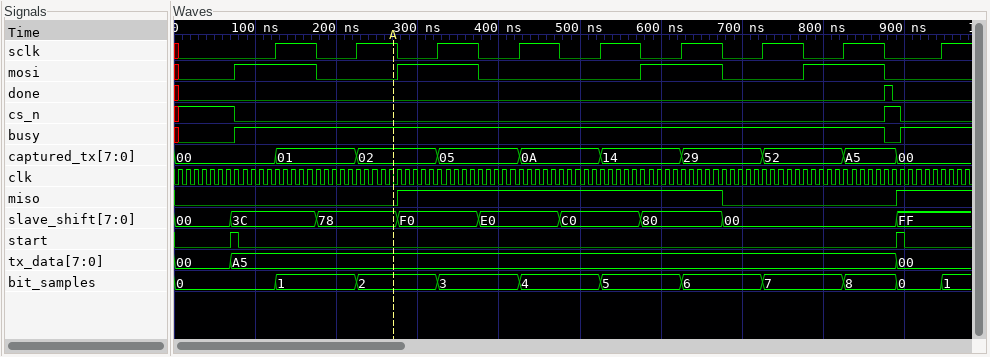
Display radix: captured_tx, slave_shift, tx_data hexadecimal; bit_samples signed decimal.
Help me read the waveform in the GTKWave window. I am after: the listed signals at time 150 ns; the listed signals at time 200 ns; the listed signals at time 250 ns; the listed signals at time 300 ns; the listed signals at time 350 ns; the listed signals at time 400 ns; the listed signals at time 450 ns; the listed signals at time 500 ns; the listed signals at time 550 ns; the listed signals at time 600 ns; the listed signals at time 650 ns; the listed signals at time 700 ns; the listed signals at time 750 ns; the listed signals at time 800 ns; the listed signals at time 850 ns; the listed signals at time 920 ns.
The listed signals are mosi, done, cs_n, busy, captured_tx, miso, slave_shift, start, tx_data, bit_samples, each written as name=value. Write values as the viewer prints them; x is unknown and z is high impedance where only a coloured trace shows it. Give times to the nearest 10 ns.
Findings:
mosi=1, done=0, cs_n=0, busy=1, captured_tx=01, miso=0, slave_shift=3C, start=0, tx_data=A5, bit_samples=1
mosi=0, done=0, cs_n=0, busy=1, captured_tx=01, miso=0, slave_shift=78, start=0, tx_data=A5, bit_samples=1
mosi=0, done=0, cs_n=0, busy=1, captured_tx=02, miso=0, slave_shift=78, start=0, tx_data=A5, bit_samples=2
mosi=1, done=0, cs_n=0, busy=1, captured_tx=02, miso=1, slave_shift=F0, start=0, tx_data=A5, bit_samples=2
mosi=1, done=0, cs_n=0, busy=1, captured_tx=05, miso=1, slave_shift=F0, start=0, tx_data=A5, bit_samples=3
mosi=0, done=0, cs_n=0, busy=1, captured_tx=05, miso=1, slave_shift=E0, start=0, tx_data=A5, bit_samples=3
mosi=0, done=0, cs_n=0, busy=1, captured_tx=0A, miso=1, slave_shift=E0, start=0, tx_data=A5, bit_samples=4
mosi=0, done=0, cs_n=0, busy=1, captured_tx=0A, miso=1, slave_shift=C0, start=0, tx_data=A5, bit_samples=4
mosi=0, done=0, cs_n=0, busy=1, captured_tx=14, miso=1, slave_shift=C0, start=0, tx_data=A5, bit_samples=5
mosi=1, done=0, cs_n=0, busy=1, captured_tx=14, miso=1, slave_shift=80, start=0, tx_data=A5, bit_samples=5
mosi=1, done=0, cs_n=0, busy=1, captured_tx=29, miso=1, slave_shift=80, start=0, tx_data=A5, bit_samples=6
mosi=0, done=0, cs_n=0, busy=1, captured_tx=29, miso=0, slave_shift=00, start=0, tx_data=A5, bit_samples=6
mosi=0, done=0, cs_n=0, busy=1, captured_tx=52, miso=0, slave_shift=00, start=0, tx_data=A5, bit_samples=7
mosi=1, done=0, cs_n=0, busy=1, captured_tx=52, miso=0, slave_shift=00, start=0, tx_data=A5, bit_samples=7
mosi=1, done=0, cs_n=0, busy=1, captured_tx=A5, miso=0, slave_shift=00, start=0, tx_data=A5, bit_samples=8
mosi=0, done=0, cs_n=0, busy=1, captured_tx=00, miso=1, slave_shift=FF, start=0, tx_data=00, bit_samples=0
